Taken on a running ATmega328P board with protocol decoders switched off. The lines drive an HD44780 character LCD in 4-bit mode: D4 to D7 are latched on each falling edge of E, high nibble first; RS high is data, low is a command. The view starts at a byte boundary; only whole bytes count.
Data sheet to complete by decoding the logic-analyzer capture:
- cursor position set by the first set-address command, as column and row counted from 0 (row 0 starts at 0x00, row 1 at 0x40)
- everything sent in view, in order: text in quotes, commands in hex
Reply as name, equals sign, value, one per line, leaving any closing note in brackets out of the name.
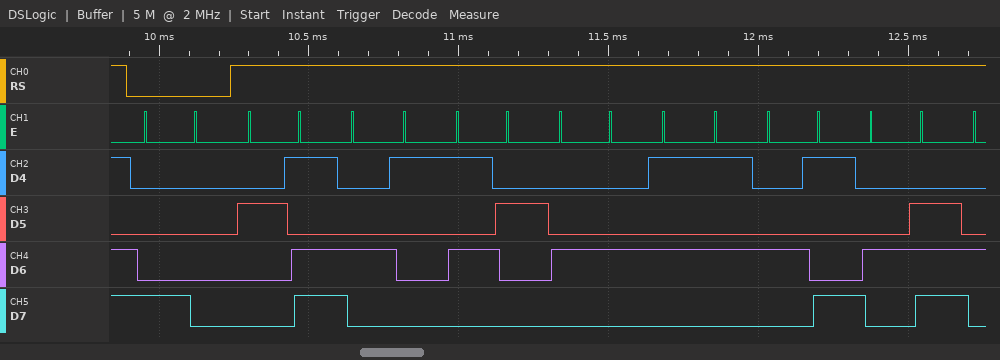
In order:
cursor position set by the first set-address command, as column and row counted from 0 = column 0, row 0
everything sent in view, in order: text in quotes, commands in hex = 0x80 "-ARDUIN"
